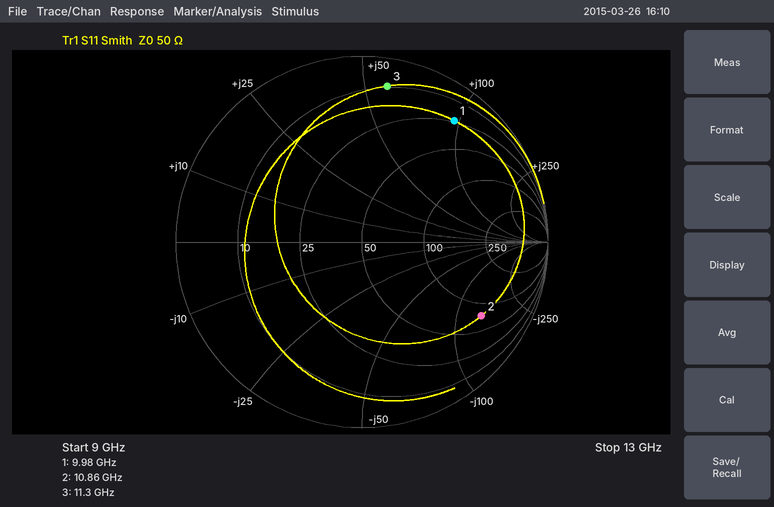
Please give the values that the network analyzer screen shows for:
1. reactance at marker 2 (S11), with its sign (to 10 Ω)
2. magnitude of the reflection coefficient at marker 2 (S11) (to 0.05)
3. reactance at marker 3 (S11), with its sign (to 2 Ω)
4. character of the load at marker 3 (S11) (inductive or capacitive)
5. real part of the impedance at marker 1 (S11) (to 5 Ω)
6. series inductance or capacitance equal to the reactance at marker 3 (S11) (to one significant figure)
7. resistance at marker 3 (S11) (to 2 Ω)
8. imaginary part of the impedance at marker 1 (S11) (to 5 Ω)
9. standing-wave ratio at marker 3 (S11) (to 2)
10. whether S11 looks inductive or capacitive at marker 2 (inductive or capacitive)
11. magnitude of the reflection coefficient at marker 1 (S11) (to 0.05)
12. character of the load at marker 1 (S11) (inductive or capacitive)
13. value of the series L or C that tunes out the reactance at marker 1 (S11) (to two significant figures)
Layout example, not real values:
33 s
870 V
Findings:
-140 Ω
0.75
+58 Ω
inductive
25 Ω
800 pH
10 Ω
+95 Ω
12
capacitive
0.80
inductive
170 fF
